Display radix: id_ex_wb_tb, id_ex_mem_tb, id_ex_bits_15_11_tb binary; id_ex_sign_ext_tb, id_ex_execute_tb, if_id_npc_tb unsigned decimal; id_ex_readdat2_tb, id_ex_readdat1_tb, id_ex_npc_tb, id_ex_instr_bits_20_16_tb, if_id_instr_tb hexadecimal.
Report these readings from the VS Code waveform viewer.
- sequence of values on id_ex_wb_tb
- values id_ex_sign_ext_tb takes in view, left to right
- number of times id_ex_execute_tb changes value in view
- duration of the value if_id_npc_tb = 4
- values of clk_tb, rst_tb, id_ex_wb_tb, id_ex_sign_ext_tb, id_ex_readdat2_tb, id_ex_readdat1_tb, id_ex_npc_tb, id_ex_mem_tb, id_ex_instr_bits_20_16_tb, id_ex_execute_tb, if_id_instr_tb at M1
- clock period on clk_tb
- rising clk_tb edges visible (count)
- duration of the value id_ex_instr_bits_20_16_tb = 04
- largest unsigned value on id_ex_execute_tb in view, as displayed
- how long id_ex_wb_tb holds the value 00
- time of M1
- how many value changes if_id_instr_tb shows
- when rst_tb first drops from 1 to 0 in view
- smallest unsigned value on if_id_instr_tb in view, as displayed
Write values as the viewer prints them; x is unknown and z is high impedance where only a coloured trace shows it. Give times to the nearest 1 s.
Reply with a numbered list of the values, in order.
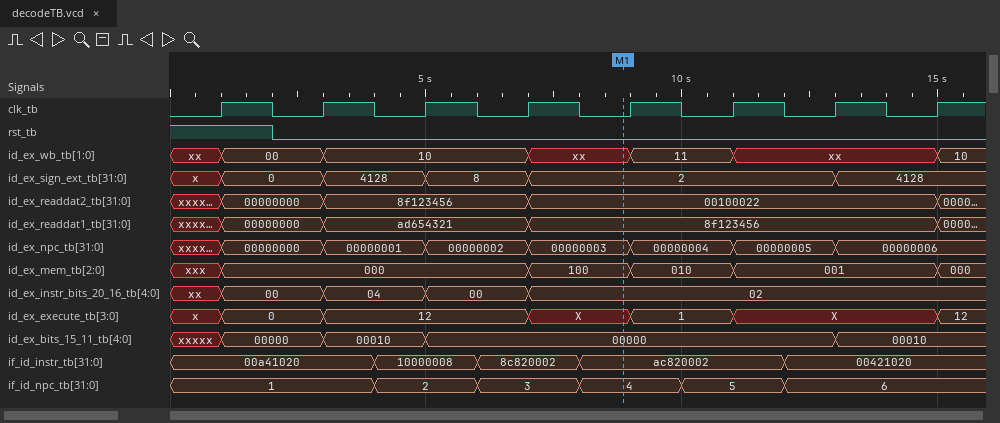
1. xx, 00, 10, xx, 11, xx, 10
2. x, 0, 4128, 8, 2, 4128
3. 6
4. 2 s
5. clk_tb=0, rst_tb=0, id_ex_wb_tb=xx, id_ex_sign_ext_tb=2, id_ex_readdat2_tb=00100022, id_ex_readdat1_tb=8f123456, id_ex_npc_tb=00000003, id_ex_mem_tb=100, id_ex_instr_bits_20_16_tb=02, id_ex_execute_tb=X, if_id_instr_tb=ac820002
6. 2 s
7. 8
8. 2 s
9. 12
10. 2 s
11. 9 s
12. 4
13. 2 s
14. 00421020
